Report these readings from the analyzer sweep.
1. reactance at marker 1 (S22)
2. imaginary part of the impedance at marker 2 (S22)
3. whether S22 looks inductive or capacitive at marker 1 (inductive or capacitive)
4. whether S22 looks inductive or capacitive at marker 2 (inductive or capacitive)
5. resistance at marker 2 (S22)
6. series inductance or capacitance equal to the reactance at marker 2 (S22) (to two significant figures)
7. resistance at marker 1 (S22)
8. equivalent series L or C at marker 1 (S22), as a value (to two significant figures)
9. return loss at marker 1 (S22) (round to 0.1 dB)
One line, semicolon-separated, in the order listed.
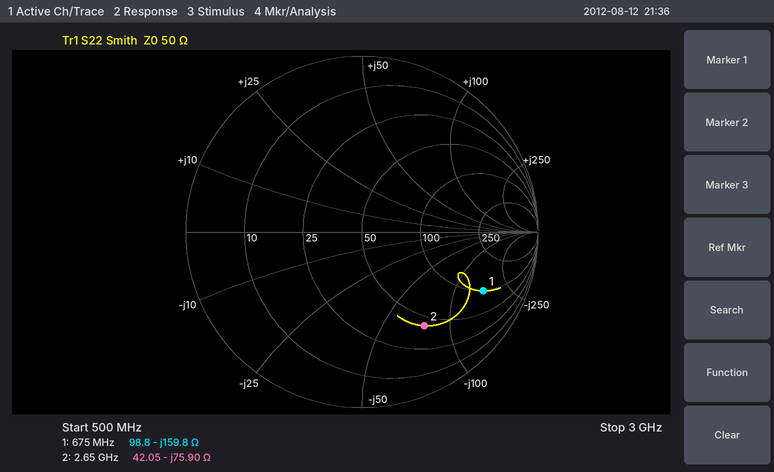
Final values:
-159.8 Ω; -75.90 Ω; capacitive; capacitive; 42.05 Ω; 790 fF; 98.8 Ω; 1.5 pF; 2.3 dB
